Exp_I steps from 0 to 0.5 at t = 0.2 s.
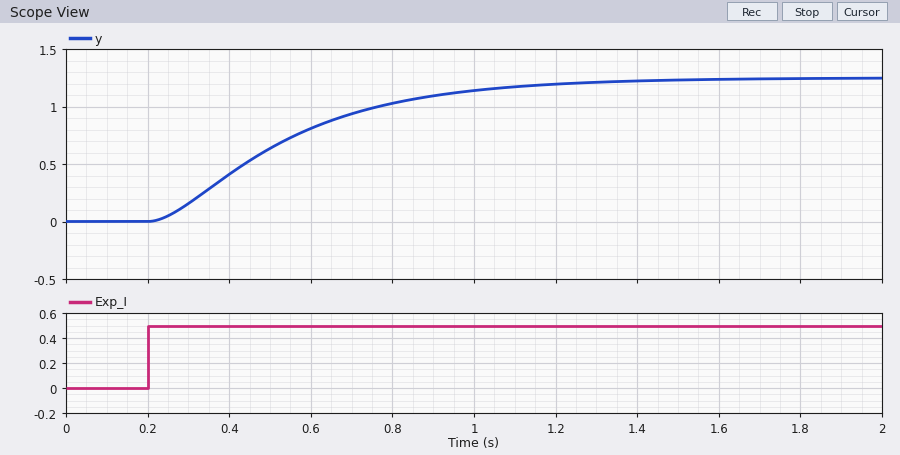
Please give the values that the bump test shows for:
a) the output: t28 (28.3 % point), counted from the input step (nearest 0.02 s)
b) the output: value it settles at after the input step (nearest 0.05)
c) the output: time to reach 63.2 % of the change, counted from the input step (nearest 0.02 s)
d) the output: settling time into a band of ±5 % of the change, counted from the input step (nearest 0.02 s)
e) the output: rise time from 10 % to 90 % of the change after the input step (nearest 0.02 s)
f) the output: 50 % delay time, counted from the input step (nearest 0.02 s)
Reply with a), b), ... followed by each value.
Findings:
a) 0.18 s
b) 1.25
c) 0.38 s
d) 0.96 s
e) 0.68 s
f) 0.30 s
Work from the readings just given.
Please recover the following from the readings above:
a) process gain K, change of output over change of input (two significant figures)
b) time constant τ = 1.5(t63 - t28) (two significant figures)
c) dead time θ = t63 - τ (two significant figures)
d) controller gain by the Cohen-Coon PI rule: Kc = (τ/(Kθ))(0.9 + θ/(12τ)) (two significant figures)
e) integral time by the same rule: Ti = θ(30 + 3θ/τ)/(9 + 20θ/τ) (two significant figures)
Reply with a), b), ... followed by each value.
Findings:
a) 2.5
b) 0.30 s
c) 0.080 s
d) 1.4
e) 0.17 s
